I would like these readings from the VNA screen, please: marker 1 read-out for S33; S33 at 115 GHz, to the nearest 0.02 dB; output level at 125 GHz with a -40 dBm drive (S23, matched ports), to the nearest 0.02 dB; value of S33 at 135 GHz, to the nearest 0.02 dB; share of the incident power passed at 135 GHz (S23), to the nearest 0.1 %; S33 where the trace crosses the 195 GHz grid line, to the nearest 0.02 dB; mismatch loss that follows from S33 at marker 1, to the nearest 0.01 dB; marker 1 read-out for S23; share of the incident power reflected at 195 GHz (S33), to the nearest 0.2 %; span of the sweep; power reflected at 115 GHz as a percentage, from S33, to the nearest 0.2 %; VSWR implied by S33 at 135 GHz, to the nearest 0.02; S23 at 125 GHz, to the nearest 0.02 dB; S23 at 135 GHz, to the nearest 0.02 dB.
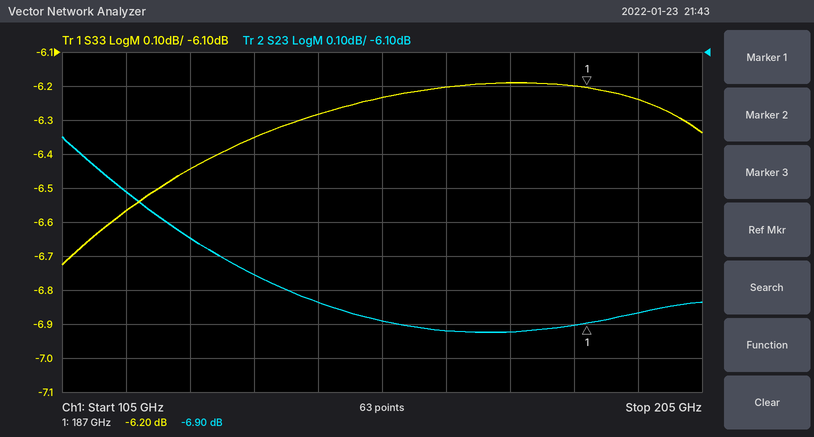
-6.20 dB
-6.56 dB
-46.64 dBm
-6.36 dB
21.1 %
-6.24 dB
1.19 dB
-6.90 dB
23.8 %
100 GHz
22.0 %
2.86
-6.64 dB
-6.76 dB
